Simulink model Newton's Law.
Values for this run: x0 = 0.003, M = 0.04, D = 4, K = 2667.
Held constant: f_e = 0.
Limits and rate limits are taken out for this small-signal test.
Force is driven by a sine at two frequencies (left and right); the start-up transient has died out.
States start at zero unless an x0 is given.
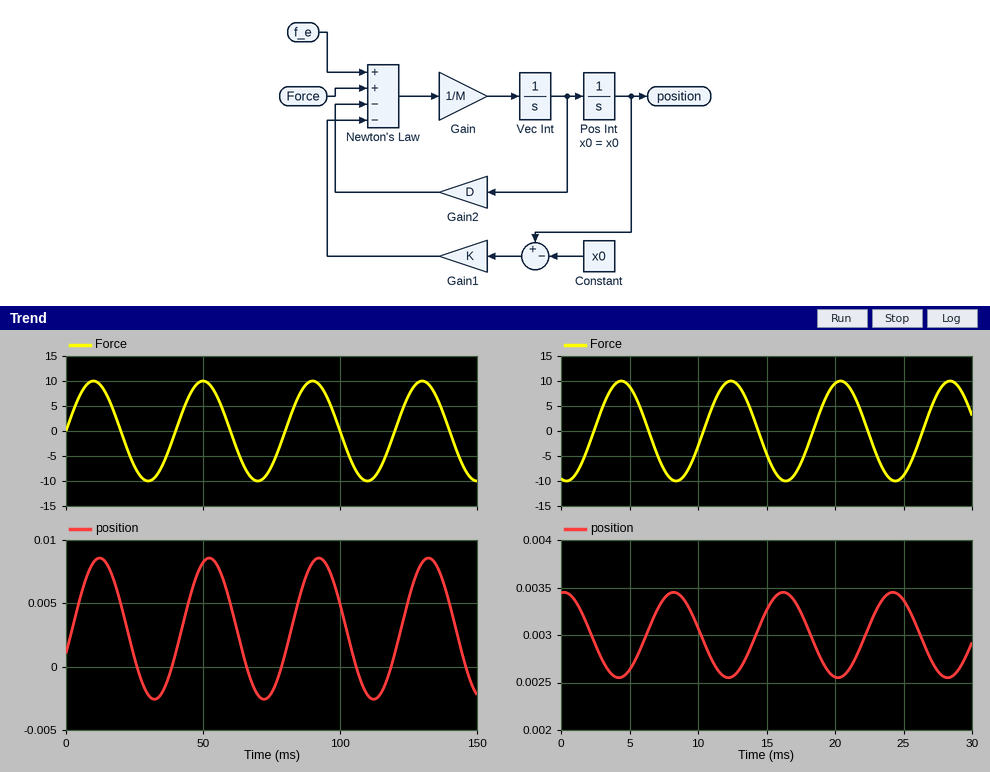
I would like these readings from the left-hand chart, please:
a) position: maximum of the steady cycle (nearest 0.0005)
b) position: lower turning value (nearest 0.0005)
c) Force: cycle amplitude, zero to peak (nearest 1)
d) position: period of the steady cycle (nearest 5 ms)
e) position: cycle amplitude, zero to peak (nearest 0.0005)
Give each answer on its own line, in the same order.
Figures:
0.0085
-0.0025
10
40 ms
0.0055
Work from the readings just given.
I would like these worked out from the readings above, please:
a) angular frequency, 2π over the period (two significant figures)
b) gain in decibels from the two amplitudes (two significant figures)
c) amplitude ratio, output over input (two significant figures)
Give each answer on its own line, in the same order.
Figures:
0.16 rad/ms
-65 dB
0.00055
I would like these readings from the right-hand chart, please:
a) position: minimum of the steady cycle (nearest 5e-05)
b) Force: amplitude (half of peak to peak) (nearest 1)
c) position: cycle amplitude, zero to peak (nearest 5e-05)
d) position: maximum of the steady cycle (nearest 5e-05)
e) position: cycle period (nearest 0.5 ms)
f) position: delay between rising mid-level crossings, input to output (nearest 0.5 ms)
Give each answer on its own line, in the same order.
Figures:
0.00255
10
0.00045
0.00345
8.0 ms
4.0 ms
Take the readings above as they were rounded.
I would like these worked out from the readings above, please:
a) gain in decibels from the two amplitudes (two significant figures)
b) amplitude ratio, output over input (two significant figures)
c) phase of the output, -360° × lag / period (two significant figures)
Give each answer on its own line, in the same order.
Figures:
-87 dB
0.000045
-180°
